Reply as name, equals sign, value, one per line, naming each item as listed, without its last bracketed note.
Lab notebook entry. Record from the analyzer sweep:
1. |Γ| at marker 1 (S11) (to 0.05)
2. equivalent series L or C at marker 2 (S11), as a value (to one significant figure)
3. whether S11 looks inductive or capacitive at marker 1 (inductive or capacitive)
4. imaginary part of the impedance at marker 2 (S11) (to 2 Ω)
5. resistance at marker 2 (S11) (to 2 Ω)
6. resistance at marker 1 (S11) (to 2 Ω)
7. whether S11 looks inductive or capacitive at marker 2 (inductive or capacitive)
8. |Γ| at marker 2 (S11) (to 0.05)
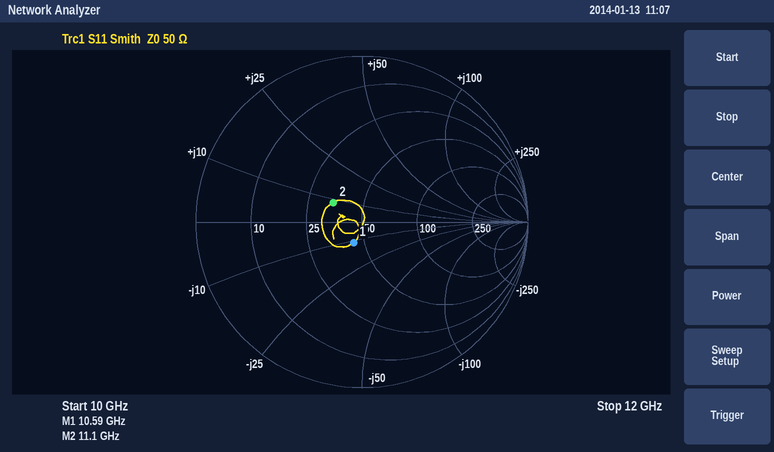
|Γ| at marker 1 (S11) = 0.15
equivalent series L or C at marker 2 (S11), as a value = 100 pH
whether S11 looks inductive or capacitive at marker 1 = capacitive
imaginary part of the impedance at marker 2 (S11) = +8 Ω
resistance at marker 2 (S11) = 34 Ω
resistance at marker 1 (S11) = 44 Ω
whether S11 looks inductive or capacitive at marker 2 = inductive
|Γ| at marker 2 (S11) = 0.20
